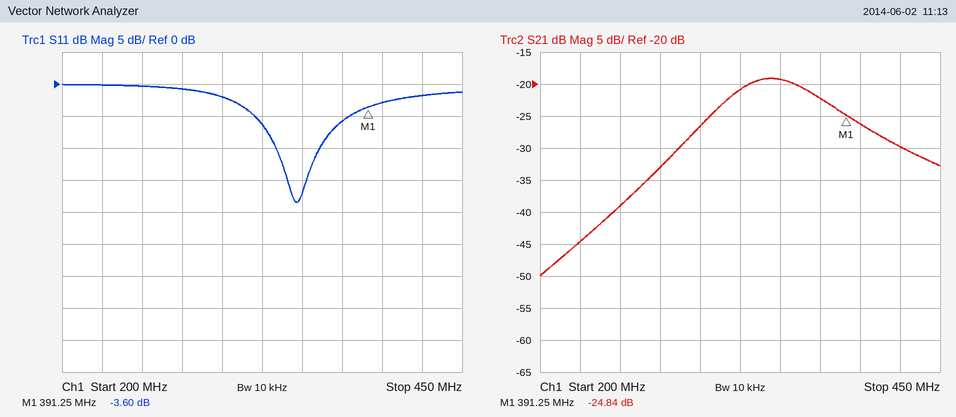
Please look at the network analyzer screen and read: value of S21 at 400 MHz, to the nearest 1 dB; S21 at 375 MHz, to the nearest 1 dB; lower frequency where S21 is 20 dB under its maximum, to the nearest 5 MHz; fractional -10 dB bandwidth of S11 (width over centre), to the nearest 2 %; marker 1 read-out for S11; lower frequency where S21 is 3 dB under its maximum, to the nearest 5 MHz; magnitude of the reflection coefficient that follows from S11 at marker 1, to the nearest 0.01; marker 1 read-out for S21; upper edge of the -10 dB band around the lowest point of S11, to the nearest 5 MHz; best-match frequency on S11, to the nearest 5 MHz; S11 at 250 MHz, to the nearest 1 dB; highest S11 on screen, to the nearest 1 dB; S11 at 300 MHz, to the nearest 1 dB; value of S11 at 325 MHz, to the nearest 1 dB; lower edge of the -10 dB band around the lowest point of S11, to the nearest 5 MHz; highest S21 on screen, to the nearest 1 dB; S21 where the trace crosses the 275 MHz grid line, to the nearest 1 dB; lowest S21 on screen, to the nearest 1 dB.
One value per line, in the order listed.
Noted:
-26 dB
-22 dB
250 MHz
8 %
-3.60 dB
320 MHz
0.66
-24.84 dB
360 MHz
345 MHz
0 dB
0 dB
-2 dB
-6 dB
335 MHz
-19 dB
-33 dB
-50 dB
